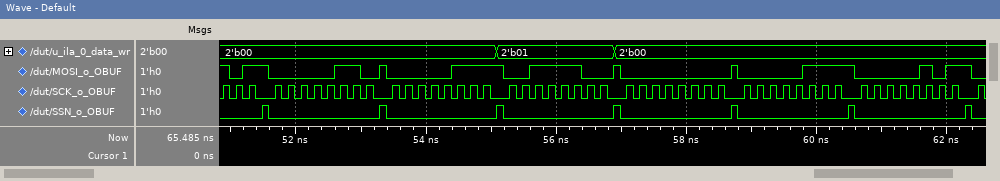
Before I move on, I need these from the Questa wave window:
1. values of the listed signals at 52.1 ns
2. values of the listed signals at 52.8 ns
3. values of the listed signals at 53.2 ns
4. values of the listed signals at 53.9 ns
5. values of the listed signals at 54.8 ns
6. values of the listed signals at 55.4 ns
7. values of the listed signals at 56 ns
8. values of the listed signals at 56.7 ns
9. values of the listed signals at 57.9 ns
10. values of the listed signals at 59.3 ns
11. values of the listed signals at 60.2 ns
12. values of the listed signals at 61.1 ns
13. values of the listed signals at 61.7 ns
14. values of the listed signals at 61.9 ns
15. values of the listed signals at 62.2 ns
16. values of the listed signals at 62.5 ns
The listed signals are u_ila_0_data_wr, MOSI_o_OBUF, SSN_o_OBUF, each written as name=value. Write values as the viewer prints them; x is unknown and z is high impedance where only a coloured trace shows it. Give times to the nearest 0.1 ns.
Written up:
u_ila_0_data_wr=2'b00, MOSI_o_OBUF=0, SSN_o_OBUF=0
u_ila_0_data_wr=2'b00, MOSI_o_OBUF=1, SSN_o_OBUF=0
u_ila_0_data_wr=2'b00, MOSI_o_OBUF=0, SSN_o_OBUF=0
u_ila_0_data_wr=2'b00, MOSI_o_OBUF=0, SSN_o_OBUF=0
u_ila_0_data_wr=2'b00, MOSI_o_OBUF=1, SSN_o_OBUF=0
u_ila_0_data_wr=2'b01, MOSI_o_OBUF=0, SSN_o_OBUF=0
u_ila_0_data_wr=2'b01, MOSI_o_OBUF=1, SSN_o_OBUF=0
u_ila_0_data_wr=2'b01, MOSI_o_OBUF=0, SSN_o_OBUF=0
u_ila_0_data_wr=2'b00, MOSI_o_OBUF=0, SSN_o_OBUF=0
u_ila_0_data_wr=2'b00, MOSI_o_OBUF=0, SSN_o_OBUF=0
u_ila_0_data_wr=2'b00, MOSI_o_OBUF=1, SSN_o_OBUF=0
u_ila_0_data_wr=2'b00, MOSI_o_OBUF=0, SSN_o_OBUF=0
u_ila_0_data_wr=2'b00, MOSI_o_OBUF=1, SSN_o_OBUF=0
u_ila_0_data_wr=2'b00, MOSI_o_OBUF=0, SSN_o_OBUF=0
u_ila_0_data_wr=2'b00, MOSI_o_OBUF=1, SSN_o_OBUF=0
u_ila_0_data_wr=2'b00, MOSI_o_OBUF=0, SSN_o_OBUF=0
